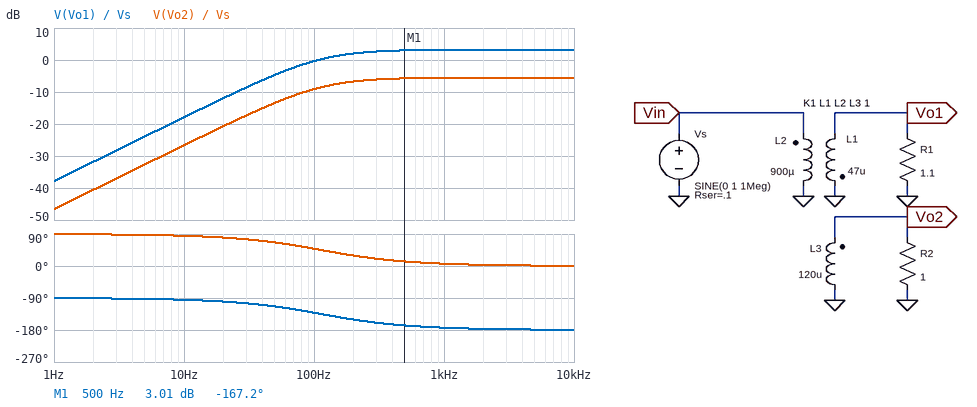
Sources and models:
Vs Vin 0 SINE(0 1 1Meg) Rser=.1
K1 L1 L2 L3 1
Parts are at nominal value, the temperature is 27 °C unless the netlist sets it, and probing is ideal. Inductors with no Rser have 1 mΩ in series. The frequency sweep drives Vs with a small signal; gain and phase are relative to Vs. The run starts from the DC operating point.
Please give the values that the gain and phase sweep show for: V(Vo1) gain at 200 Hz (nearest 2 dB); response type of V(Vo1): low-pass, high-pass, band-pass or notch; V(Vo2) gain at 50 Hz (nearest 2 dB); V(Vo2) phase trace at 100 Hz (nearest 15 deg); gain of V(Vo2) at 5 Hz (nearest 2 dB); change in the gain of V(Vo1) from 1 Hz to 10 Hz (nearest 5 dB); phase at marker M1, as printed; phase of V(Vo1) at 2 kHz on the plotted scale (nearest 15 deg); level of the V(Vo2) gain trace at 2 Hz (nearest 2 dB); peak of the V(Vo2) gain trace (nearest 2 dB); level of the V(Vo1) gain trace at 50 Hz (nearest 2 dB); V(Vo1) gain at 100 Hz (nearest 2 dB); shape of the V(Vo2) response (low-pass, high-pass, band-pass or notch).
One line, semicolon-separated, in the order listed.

2 dB; high-pass; -14 dB; 45 deg; -32 dB; 20 dB; -167.2 deg; -180 deg; -40 dB; -6 dB; -4 dB; 0 dB; high-pass
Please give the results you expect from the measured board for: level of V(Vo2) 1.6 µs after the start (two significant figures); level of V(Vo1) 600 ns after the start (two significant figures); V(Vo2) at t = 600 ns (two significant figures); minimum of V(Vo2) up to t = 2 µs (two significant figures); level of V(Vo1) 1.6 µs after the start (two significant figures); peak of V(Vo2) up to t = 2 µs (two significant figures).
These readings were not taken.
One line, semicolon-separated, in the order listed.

-310 mV; 850 mV; -310 mV; -530 mV; 850 mV; 530 mV
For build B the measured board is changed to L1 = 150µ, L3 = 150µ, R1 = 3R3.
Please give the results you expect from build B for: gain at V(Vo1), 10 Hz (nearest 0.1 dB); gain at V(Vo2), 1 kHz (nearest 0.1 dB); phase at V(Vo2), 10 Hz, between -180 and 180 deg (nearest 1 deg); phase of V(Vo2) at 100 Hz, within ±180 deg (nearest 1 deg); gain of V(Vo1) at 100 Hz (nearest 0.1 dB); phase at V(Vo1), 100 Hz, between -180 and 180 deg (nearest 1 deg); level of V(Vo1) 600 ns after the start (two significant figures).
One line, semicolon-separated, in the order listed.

-12.9 dB; -2.2 dB; 83 deg; 40 deg; 3.3 dB; -140 deg; 1.1 V
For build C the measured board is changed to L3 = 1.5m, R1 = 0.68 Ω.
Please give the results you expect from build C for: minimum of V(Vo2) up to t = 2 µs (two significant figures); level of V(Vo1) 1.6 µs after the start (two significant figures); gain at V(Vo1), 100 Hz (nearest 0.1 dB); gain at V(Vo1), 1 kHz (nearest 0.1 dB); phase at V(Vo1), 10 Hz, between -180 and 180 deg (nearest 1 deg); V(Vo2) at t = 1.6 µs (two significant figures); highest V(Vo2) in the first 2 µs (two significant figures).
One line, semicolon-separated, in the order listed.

-800 mV; 360 mV; -5.1 dB; -4.2 dB; -102 deg; -470 mV; 800 mV
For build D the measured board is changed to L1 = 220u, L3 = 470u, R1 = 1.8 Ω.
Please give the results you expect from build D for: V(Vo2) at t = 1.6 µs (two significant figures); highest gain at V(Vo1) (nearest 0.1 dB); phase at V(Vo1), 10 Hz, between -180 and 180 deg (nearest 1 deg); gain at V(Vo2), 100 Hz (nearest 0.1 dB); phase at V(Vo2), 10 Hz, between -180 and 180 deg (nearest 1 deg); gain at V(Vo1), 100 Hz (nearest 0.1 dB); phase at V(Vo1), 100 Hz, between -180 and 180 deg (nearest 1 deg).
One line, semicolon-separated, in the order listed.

-590 mV; 2.9 dB; -101 deg; -0.9 dB; 79 deg; 1.9 dB; -153 deg
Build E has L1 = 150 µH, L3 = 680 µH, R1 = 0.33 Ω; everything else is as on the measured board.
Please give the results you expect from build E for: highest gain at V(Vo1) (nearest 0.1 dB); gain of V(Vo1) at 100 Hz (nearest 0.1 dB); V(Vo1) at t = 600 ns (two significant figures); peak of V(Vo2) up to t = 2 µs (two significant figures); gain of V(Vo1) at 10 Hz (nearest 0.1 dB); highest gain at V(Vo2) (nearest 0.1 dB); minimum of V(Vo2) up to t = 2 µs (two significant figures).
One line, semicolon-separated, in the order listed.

-2.6 dB; -3.0 dB; 440 mV; 650 mV; -13.2 dB; -3.8 dB; -650 mV
